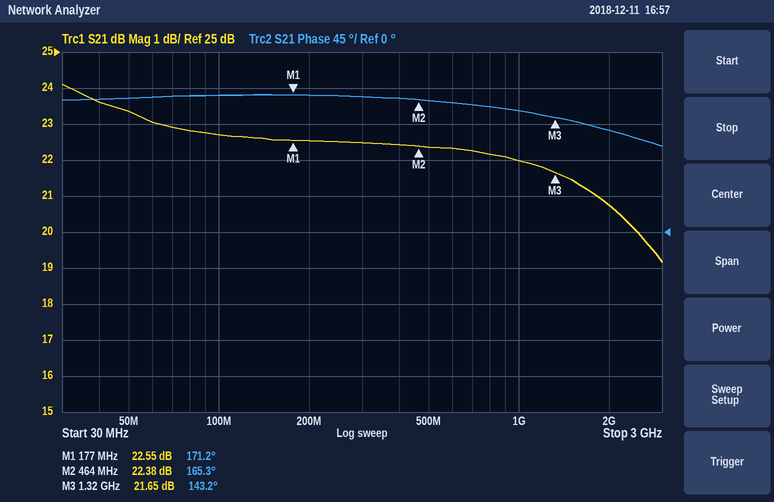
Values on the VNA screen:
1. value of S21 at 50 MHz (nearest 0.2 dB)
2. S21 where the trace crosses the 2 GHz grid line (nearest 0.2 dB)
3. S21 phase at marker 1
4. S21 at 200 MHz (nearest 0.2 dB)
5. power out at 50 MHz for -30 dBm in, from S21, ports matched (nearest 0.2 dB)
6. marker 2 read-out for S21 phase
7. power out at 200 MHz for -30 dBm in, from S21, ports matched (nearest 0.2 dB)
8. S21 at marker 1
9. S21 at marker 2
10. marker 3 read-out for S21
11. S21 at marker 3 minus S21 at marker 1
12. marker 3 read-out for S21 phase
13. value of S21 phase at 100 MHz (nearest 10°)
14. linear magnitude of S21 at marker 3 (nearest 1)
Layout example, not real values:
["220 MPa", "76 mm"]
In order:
["23.4 dB", "20.8 dB", "171.2°", "22.6 dB", "-6.6 dBm", "165.3°", "-7.4 dBm", "22.55 dB", "22.38 dB", "21.65 dB", "-0.90 dB", "143.2°", "170°", "12"]
